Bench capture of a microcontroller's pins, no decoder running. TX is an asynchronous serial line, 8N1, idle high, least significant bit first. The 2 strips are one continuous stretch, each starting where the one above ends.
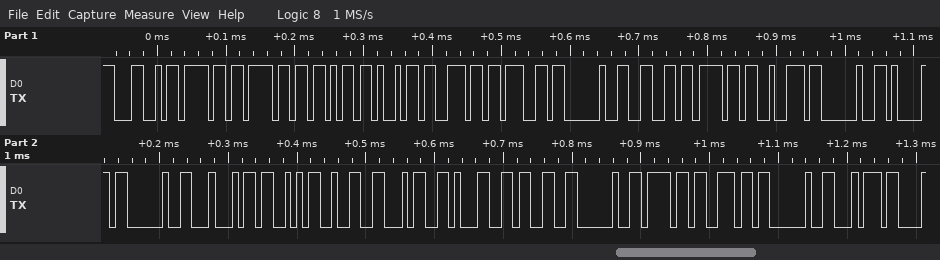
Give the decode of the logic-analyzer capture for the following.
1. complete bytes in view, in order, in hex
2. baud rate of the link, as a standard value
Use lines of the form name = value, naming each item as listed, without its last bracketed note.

complete bytes in view, in order, in hex = 0x4C 0x6F 0x6F 0x6B 0x69 0x6E 0x67 0x20 0x66 0x6F 0x72 0x20 0x61 0x20 0x44 0x53 0x32 0x34 0x31 0x33 0x20 0x6F 0x6E 0x20 0x74
baud rate of the link, as a standard value = 115200 baud
